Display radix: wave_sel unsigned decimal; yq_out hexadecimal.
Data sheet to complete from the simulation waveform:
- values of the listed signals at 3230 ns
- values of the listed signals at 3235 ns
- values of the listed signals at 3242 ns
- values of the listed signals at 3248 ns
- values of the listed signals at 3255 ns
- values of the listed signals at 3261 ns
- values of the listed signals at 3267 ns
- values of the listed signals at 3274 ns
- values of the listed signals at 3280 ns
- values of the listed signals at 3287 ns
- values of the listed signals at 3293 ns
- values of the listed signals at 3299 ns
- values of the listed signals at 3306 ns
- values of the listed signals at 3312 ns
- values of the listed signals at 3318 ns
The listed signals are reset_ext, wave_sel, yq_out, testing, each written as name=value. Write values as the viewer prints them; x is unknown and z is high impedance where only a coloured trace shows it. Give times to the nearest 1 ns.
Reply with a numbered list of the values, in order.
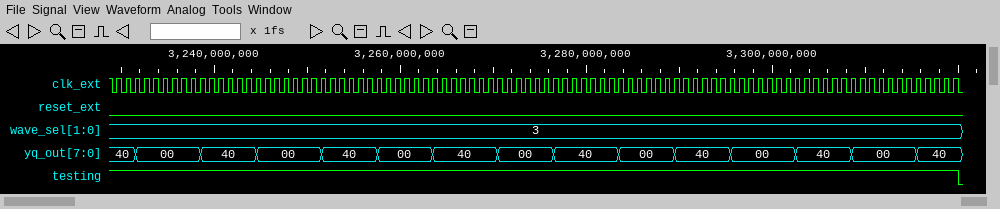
1. reset_ext=0, wave_sel=3, yq_out=40, testing=1
2. reset_ext=0, wave_sel=3, yq_out=00, testing=1
3. reset_ext=0, wave_sel=3, yq_out=40, testing=1
4. reset_ext=0, wave_sel=3, yq_out=00, testing=1
5. reset_ext=0, wave_sel=3, yq_out=40, testing=1
6. reset_ext=0, wave_sel=3, yq_out=00, testing=1
7. reset_ext=0, wave_sel=3, yq_out=40, testing=1
8. reset_ext=0, wave_sel=3, yq_out=00, testing=1
9. reset_ext=0, wave_sel=3, yq_out=40, testing=1
10. reset_ext=0, wave_sel=3, yq_out=00, testing=1
11. reset_ext=0, wave_sel=3, yq_out=40, testing=1
12. reset_ext=0, wave_sel=3, yq_out=00, testing=1
13. reset_ext=0, wave_sel=3, yq_out=40, testing=1
14. reset_ext=0, wave_sel=3, yq_out=00, testing=1
15. reset_ext=0, wave_sel=3, yq_out=40, testing=1
